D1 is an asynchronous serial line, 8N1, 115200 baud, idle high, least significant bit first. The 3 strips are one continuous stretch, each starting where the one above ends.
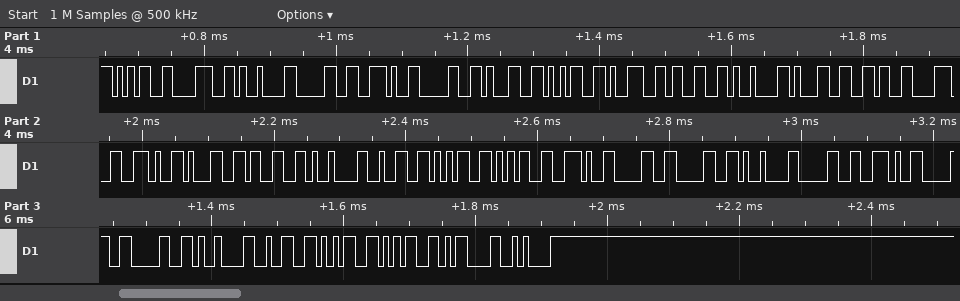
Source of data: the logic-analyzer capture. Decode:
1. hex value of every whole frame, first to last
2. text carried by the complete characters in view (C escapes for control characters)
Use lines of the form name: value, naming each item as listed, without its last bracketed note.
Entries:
hex value of every whole frame, first to last: 0x35 0x38 0x09 0x30 0x2E 0x30 0x31 0x35 0x39 0x33 0x09 0x31 0x36 0x38 0x2E 0x31 0x33 0x09 0x32 0x35 0x35 0x2E 0x30 0x30 0x09 0x30 0x2E 0x30 0x30 0x09 0x32 0x35 0x35 0x0D 0x0A
text carried by the complete characters in view: "58\t0.01593\t168.13\t255.00\t0.00\t255\r\n"
